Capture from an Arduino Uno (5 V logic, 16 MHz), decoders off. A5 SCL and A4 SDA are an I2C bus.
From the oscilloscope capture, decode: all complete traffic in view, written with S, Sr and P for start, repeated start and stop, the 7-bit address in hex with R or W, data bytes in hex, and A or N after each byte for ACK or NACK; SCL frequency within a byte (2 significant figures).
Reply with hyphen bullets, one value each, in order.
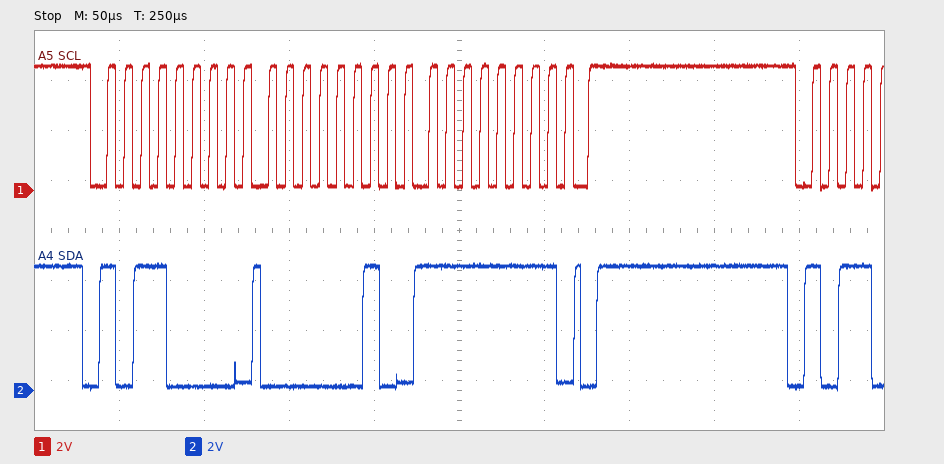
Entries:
- S 58W A 02 A FF A P
- 100 kHz
